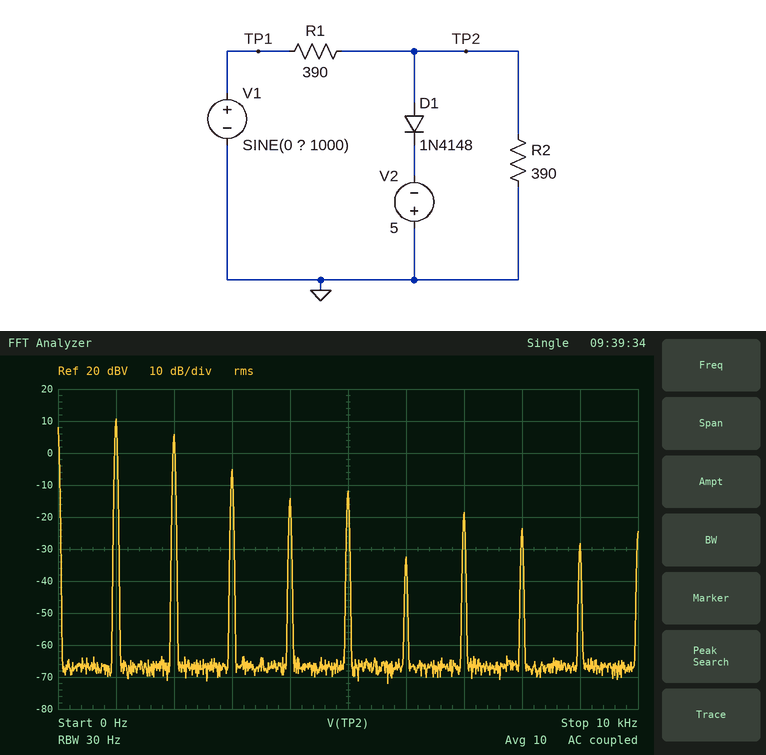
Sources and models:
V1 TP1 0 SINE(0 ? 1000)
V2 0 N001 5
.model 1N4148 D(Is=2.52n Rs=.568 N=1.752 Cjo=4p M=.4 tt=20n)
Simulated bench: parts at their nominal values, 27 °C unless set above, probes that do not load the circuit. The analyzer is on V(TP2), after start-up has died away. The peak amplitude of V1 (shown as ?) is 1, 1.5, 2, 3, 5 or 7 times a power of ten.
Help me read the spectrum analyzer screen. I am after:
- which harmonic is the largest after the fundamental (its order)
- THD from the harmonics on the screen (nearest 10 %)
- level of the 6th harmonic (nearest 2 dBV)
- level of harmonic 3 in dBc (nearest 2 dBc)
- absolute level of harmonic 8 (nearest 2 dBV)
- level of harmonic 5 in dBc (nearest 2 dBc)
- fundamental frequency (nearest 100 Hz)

2
60 %
-32 dBV
-16 dBc
-24 dBV
-22 dBc
1.0 kHz
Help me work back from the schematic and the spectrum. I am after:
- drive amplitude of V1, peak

30 V
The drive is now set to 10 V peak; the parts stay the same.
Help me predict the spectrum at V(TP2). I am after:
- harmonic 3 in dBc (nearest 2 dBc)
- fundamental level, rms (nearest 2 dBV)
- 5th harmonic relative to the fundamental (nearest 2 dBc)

-6 dBc
-16 dBV
-12 dBc
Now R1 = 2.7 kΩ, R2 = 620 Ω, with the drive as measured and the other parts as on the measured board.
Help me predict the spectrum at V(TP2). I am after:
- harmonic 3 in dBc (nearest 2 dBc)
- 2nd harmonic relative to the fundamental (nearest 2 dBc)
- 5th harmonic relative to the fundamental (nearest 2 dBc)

-6 dBc
-2 dBc
-14 dBc
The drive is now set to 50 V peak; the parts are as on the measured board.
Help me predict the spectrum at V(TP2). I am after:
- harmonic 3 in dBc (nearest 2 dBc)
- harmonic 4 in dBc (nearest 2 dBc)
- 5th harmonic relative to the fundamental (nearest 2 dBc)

-22 dBc
-22 dBc
-26 dBc
